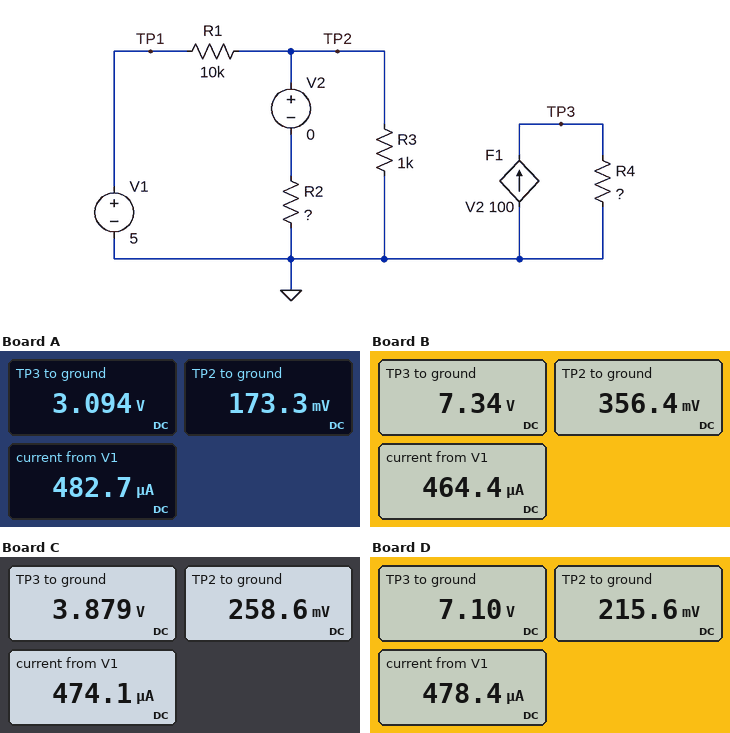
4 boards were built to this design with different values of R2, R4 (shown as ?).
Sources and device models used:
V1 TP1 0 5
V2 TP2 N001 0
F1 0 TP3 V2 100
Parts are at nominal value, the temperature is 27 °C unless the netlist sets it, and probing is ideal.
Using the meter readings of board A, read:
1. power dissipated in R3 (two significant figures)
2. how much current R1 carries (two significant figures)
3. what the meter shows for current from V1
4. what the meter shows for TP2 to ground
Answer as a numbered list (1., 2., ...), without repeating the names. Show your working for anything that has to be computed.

1. (173.3 mV)^2 / 1 kΩ = 30 µW
2. (5 V - 173.3 mV) / 10 kΩ = 480 µA
3. 482.7 µA
4. 173.3 mV
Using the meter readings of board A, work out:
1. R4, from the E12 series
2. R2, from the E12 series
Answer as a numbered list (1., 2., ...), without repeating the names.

1. 100 Ω
2. 560 Ω
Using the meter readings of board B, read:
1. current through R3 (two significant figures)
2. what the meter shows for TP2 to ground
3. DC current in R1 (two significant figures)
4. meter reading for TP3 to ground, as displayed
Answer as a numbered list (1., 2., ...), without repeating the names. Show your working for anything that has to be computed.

1. (356.4 mV) / 1 kΩ = 360 µA
2. 356.4 mV
3. (5 V - 356.4 mV) / 10 kΩ = 460 µA
4. 7.34 V
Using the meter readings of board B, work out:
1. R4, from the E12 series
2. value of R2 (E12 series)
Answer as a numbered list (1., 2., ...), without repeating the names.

1. 680 Ω
2. 3.3 kΩ
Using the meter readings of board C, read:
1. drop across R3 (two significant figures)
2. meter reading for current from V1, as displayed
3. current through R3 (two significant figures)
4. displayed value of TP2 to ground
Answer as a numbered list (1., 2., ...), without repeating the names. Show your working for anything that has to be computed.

1. 258.6 mV = 260 mV
2. 474.1 µA
3. (258.6 mV) / 1 kΩ = 260 µA
4. 258.6 mV
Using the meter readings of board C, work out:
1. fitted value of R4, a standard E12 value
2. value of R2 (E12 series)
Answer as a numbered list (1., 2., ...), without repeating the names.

1. 180 Ω
2. 1.2 kΩ
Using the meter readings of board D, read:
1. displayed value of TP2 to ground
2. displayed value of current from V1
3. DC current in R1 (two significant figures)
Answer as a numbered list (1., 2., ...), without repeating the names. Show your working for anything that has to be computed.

1. 215.6 mV
2. 478.4 µA
3. (5 V - 215.6 mV) / 10 kΩ = 480 µA
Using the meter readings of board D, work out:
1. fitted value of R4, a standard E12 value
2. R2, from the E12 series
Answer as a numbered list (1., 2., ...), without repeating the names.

1. 270 Ω
2. 820 Ω
